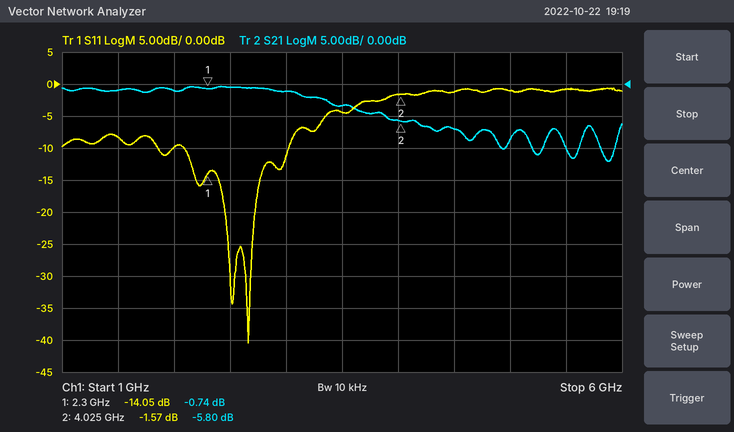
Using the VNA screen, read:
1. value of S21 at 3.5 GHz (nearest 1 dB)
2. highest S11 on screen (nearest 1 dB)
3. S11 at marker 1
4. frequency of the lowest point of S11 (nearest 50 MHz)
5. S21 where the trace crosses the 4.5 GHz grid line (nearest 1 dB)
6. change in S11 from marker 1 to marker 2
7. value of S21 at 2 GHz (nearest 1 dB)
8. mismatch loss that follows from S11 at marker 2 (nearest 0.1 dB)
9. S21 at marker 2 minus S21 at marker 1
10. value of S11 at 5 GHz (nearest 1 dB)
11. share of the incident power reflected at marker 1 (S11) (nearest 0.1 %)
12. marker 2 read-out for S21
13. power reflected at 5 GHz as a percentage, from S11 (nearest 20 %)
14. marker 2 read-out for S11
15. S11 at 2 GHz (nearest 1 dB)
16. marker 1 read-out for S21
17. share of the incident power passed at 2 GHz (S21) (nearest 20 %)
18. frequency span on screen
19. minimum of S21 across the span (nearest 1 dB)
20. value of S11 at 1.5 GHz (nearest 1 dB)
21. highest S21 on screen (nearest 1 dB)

-3 dB
-1 dB
-14.05 dB
2.65 GHz
-7 dB
12.48 dB
-1 dB
5.2 dB
-5.06 dB
-1 dB
3.9 %
-5.80 dB
80 %
-1.57 dB
-10 dB
-0.74 dB
80 %
5 GHz
-12 dB
-8 dB
0 dB
